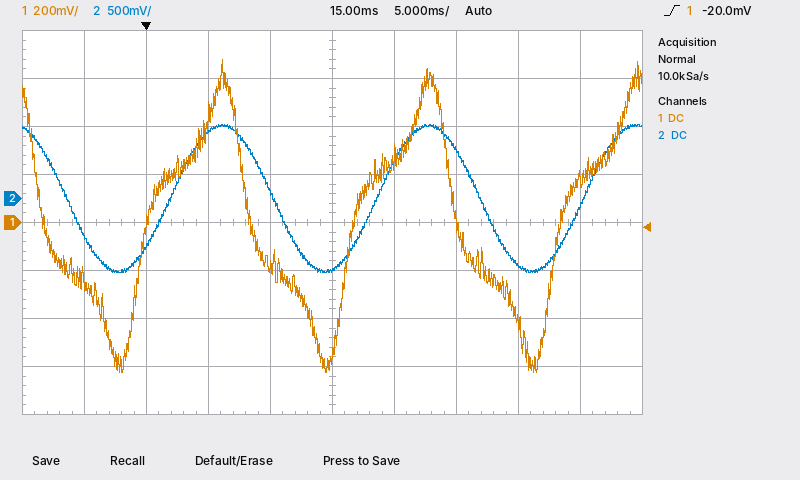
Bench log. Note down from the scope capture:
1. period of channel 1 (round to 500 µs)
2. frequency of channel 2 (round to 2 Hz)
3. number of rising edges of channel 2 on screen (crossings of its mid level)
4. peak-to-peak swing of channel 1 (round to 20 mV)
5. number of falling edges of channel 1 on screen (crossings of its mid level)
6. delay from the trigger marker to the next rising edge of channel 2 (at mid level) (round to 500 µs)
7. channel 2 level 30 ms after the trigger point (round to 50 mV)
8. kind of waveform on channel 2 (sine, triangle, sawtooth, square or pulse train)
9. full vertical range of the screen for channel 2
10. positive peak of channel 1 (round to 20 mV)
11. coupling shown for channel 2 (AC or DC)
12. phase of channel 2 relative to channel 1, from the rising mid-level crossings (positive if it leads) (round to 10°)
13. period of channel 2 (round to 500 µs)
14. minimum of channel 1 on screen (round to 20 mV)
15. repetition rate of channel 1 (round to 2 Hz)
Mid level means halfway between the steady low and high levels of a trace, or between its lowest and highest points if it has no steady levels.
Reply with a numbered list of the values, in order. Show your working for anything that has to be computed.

1. 16.5 ms
2. 1 / 16.5 ms ≈ 60.6 Hz, so 60 Hz to the nearest 2 Hz
3. 3
4. 680 mV − (-620 mV) = 1.30 V
5. 3
6. 2.0 ms
7. -700 mV
8. sine
9. 4 V
10. 680 mV
11. DC
12. -40°
13. 16.5 ms
14. -620 mV
15. 1 / 16.5 ms ≈ 60.6 Hz, so 60 Hz to the nearest 2 Hz
